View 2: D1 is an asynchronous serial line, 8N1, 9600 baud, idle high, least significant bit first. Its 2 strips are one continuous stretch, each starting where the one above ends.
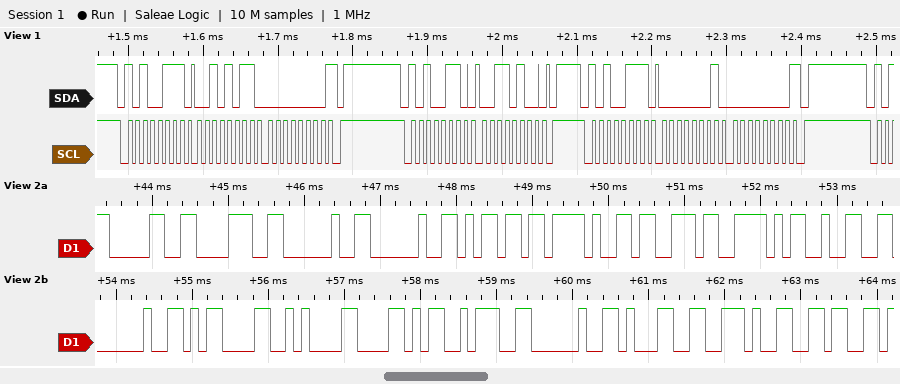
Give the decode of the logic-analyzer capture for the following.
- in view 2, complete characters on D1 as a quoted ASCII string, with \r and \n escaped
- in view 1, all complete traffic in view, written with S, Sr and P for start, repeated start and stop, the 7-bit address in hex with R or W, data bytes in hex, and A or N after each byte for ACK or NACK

"08  m/s^2 \r\nX: 1.6"
S 53R A 2B A 00 N P S 53W A 34 A P S 53R A 01 A 00 N P
